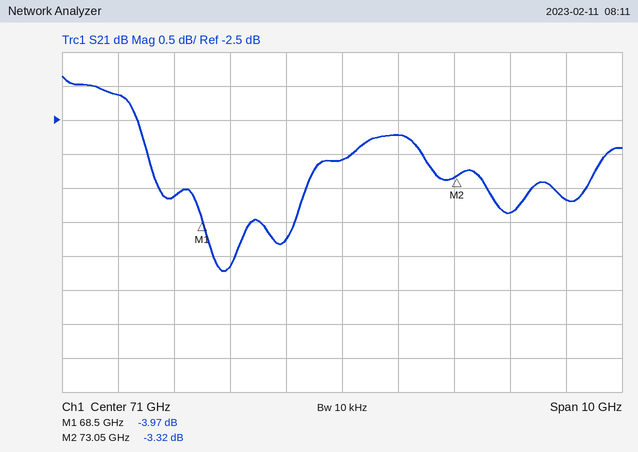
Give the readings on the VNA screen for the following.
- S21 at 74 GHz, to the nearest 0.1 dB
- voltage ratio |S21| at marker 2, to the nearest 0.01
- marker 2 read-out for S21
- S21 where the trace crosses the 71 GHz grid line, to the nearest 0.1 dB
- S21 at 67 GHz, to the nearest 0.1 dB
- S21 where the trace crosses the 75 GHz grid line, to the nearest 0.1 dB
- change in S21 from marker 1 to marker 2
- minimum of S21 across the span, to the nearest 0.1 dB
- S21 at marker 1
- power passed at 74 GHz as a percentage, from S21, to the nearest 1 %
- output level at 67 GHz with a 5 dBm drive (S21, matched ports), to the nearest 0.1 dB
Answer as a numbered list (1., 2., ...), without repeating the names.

1. -3.9 dB
2. 0.68
3. -3.32 dB
4. -3.1 dB
5. -2.1 dB
6. -3.7 dB
7. 0.65 dB
8. -4.7 dB
9. -3.97 dB
10. 41 %
11. 2.9 dBm
